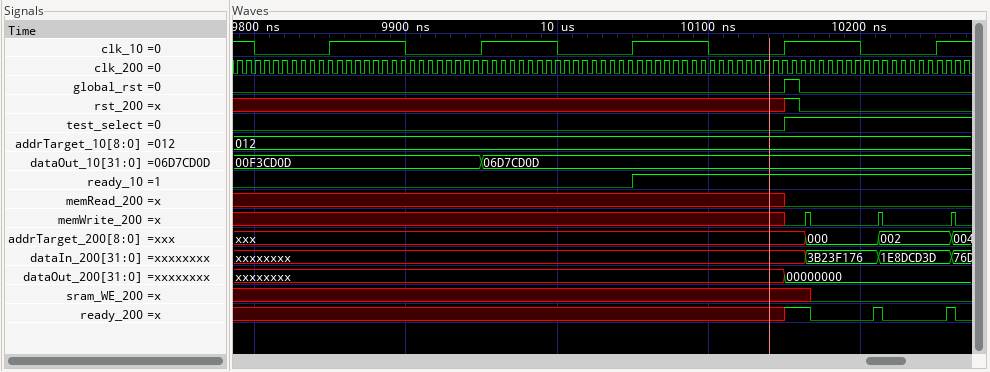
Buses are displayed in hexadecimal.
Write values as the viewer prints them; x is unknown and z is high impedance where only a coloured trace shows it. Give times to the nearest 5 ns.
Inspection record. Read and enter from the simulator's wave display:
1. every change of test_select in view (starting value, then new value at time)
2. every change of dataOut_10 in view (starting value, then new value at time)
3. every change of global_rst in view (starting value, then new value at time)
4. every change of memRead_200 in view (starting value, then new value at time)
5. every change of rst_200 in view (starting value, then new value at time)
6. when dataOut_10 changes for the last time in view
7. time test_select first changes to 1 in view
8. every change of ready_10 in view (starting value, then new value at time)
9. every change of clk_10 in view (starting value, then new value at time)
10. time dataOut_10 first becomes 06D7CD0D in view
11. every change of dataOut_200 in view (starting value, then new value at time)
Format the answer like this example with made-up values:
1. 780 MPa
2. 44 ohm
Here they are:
1. 0, 1 at 10150 ns
2. 00F3CD0D, 06D7CD0D at 9950 ns
3. 0, 1 at 10150 ns, 0 at 10160 ns
4. x, 0 at 10150 ns
5. x, 1 at 10150 ns, 0 at 10160 ns
6. 9950 ns
7. 10150 ns
8. 0, 1 at 10050 ns
9. 1, 0 at 9800 ns, 1 at 9850 ns, 0 at 9900 ns, 1 at 9950 ns, 0 at 10000 ns, 1 at 10050 ns, 0 at 10100 ns, 1 at 10150 ns, 0 at 10200 ns, 1 at 10250 ns
10. 9950 ns
11. xxxxxxxx, 00000000 at 10150 ns
